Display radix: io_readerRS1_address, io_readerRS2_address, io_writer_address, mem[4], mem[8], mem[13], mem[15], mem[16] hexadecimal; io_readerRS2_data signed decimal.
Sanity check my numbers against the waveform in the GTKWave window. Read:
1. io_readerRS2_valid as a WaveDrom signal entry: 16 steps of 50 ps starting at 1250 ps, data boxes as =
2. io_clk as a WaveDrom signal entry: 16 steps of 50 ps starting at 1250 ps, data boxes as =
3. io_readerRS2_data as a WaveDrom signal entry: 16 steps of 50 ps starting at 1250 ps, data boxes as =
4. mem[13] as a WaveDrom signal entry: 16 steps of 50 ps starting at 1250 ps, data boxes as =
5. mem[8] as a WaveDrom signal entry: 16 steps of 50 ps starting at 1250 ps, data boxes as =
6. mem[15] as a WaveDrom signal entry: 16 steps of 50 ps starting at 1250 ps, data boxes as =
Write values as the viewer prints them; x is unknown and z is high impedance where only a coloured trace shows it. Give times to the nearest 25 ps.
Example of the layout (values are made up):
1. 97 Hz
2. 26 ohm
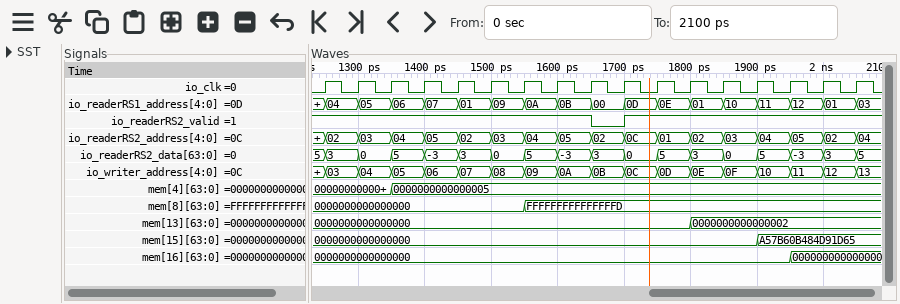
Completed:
1. {name: 'io_readerRS2_valid', wave: '1.......01......'}
2. {name: 'io_clk', wave: 'p...............'}
3. {name: 'io_readerRS2_data', wave: '================', data: '3 0 5 -3 3 0 5 -3 3 0 5 3 0 5 -3 3'}
4. {name: 'mem[13]', wave: '=..........=....', data: '0000000000000000 0000000000000002'}
5. {name: 'mem[8]', wave: '=.....=.........', data: '0000000000000000 FFFFFFFFFFFFFFFD'}
6. {name: 'mem[15]', wave: '=............=..', data: '0000000000000000 A57B60B484D91D65'}
